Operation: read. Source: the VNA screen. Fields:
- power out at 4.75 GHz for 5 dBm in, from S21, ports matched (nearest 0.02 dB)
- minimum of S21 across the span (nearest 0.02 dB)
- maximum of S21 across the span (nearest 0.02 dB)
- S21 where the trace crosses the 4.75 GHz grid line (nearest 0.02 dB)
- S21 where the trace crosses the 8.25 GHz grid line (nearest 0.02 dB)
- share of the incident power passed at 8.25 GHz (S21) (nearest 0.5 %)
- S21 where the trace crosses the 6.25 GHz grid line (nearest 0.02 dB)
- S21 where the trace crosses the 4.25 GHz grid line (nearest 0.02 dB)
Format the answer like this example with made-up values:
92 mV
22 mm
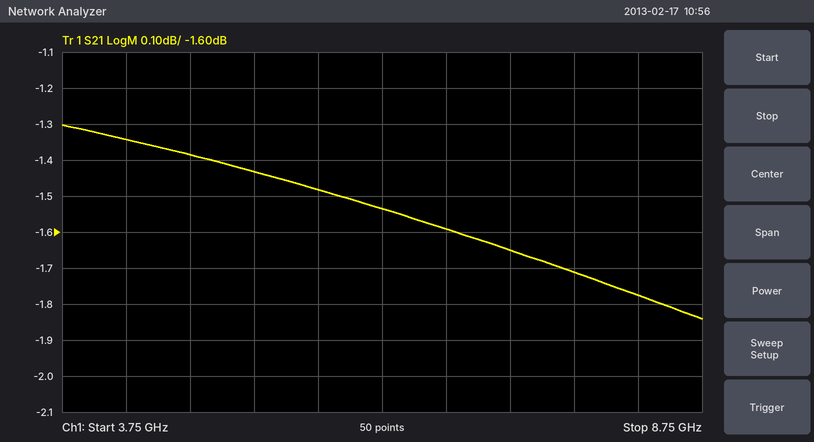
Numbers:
3.62 dBm
-1.84 dB
-1.30 dB
-1.38 dB
-1.78 dB
66.5 %
-1.54 dB
-1.34 dB
